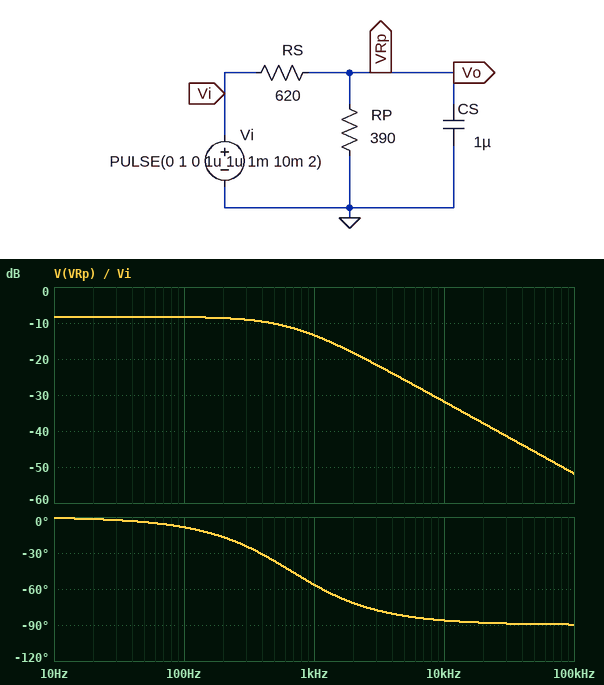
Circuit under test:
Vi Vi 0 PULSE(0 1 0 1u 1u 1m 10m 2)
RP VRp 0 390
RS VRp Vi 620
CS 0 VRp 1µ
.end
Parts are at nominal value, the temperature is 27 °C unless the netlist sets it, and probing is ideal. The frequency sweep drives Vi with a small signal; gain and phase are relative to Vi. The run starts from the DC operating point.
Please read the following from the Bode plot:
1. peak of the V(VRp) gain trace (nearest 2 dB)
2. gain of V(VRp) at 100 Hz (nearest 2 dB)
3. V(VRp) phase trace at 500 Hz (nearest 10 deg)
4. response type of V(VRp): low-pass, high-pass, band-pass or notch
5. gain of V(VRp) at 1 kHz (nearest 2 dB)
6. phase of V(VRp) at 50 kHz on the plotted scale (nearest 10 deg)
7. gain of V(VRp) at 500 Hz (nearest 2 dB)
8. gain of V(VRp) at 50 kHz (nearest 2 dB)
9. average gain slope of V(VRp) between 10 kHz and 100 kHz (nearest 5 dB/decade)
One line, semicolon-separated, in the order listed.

-8 dB; -8 dB; -40 deg; low-pass; -14 dB; -90 deg; -10 dB; -46 dB; -20 dB/decade
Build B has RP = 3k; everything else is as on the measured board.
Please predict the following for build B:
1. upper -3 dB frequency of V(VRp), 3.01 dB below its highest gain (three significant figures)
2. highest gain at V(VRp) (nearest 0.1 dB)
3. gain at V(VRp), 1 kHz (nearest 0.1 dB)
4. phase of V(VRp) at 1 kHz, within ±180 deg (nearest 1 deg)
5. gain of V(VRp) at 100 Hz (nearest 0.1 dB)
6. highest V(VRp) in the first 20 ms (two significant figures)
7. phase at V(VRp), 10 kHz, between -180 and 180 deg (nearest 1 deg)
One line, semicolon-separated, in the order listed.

310 Hz; -1.6 dB; -12.2 dB; -73 deg; -2.1 dB; 710 mV; -88 deg
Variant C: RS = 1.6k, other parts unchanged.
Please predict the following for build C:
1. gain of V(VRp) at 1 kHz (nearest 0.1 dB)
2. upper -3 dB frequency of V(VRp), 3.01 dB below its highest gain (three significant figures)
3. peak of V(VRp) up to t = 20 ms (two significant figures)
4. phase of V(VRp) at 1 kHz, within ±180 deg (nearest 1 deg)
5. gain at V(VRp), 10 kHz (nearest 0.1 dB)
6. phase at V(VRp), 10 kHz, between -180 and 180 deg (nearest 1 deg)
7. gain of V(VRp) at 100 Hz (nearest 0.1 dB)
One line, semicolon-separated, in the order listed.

-21.0 dB; 508 Hz; 190 mV; -63 deg; -40.1 dB; -87 deg; -14.3 dB
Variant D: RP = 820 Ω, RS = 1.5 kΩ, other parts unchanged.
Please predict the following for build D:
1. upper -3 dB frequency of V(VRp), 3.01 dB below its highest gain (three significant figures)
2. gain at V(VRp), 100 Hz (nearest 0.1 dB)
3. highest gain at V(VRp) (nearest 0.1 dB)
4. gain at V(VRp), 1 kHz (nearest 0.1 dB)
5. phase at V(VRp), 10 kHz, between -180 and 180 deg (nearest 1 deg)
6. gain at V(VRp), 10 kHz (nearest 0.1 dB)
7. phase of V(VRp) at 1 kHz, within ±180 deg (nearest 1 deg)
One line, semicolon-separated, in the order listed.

300 Hz; -9.5 dB; -9.0 dB; -19.9 dB; -88 deg; -39.5 dB; -73 deg
